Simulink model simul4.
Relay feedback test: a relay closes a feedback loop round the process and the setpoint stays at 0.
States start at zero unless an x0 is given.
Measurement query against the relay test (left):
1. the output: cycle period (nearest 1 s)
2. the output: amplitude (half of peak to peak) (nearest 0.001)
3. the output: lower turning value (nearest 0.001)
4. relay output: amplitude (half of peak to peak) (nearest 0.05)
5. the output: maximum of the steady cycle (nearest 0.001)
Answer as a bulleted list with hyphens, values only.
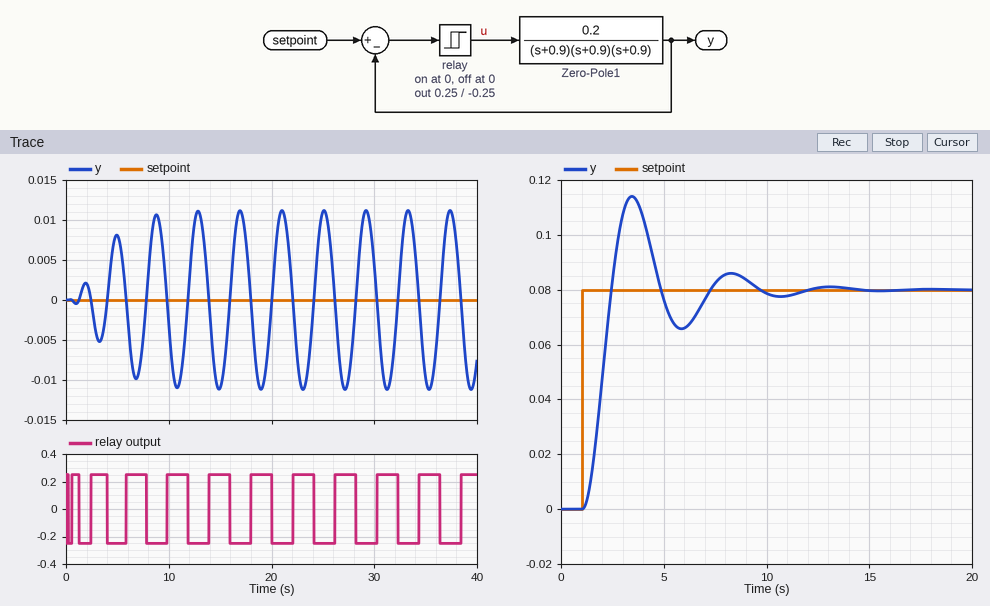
- 4 s
- 0.011
- -0.011
- 0.25
- 0.011
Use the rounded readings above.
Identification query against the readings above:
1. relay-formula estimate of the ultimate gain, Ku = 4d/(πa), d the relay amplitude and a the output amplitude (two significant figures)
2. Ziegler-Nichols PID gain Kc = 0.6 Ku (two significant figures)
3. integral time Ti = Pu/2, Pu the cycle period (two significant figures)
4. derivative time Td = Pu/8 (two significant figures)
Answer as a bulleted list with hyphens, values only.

- 29
- 17
- 2.0 s
- 0.50 s
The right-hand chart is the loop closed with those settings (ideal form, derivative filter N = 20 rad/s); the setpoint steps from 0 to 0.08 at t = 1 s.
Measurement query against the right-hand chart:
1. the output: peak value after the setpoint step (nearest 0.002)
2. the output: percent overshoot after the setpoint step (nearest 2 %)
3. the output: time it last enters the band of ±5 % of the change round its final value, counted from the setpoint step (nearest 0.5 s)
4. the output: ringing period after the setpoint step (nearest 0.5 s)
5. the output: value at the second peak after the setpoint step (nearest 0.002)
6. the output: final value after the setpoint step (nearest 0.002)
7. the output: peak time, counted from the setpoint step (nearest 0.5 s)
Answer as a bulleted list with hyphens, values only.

- 0.114
- 42 %
- 8.0 s
- 5.0 s
- 0.086
- 0.080
- 2.5 s
